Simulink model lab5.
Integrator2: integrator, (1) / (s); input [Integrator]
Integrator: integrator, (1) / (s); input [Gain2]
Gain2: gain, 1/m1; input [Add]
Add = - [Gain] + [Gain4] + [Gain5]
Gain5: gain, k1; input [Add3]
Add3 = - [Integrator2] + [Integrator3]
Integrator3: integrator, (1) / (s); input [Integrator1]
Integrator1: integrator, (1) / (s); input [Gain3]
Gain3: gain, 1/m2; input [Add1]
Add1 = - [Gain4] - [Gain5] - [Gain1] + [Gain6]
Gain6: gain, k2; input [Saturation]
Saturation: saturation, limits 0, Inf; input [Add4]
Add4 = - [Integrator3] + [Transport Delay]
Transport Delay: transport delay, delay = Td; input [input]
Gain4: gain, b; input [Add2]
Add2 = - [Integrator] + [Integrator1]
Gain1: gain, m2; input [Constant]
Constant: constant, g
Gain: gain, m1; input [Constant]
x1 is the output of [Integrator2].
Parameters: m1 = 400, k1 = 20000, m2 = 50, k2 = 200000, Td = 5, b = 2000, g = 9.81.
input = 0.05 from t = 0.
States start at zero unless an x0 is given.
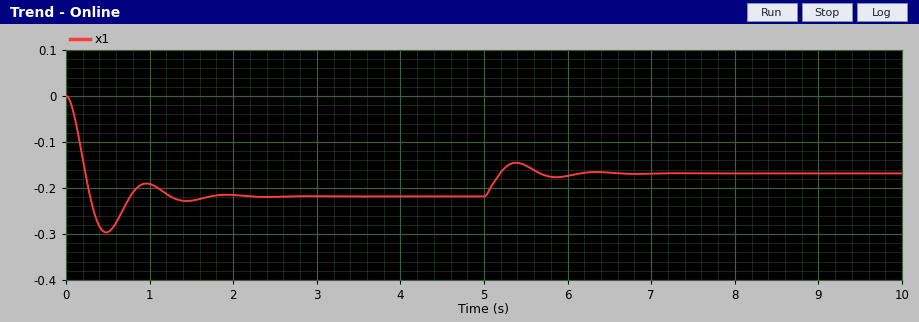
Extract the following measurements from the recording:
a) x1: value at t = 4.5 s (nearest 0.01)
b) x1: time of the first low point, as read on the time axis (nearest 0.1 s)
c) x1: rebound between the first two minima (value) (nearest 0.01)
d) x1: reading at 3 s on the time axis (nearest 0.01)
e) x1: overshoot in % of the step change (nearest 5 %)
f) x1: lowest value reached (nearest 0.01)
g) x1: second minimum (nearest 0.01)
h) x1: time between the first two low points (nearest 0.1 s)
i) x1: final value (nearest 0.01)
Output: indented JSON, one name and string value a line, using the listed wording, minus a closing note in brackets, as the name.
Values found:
{
  "x1: value at t = 4.5 s": "-0.22",
  "x1: time of the first low point, as read on the time axis": "0.5 s",
  "x1: rebound between the first two minima (value)": "-0.19",
  "x1: reading at 3 s on the time axis": "-0.22",
  "x1: overshoot in % of the step change": "75 %",
  "x1: lowest value reached": "-0.30",
  "x1: second minimum": "-0.23",
  "x1: time between the first two low points": "1.0 s",
  "x1: final value": "-0.17"
}
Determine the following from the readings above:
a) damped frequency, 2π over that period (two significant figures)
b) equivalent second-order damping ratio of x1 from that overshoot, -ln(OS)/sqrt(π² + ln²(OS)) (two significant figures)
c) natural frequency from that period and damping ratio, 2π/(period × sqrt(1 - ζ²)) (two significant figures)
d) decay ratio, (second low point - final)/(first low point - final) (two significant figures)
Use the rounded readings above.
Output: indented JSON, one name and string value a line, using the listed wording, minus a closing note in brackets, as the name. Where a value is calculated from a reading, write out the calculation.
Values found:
{
  "damped frequency, 2π over that period": "2π / 1 = 6.3 rad/s",
  "equivalent second-order damping ratio of x1 from that overshoot, -ln(OS)/sqrt(π² + ln²(OS))": "ln(0.75) = -0.288; 0.288 / sqrt(9.870 + 0.083) = 0.091",
  "natural frequency from that period and damping ratio, 2π/(period × sqrt(1 - ζ²))": "2π / (1 × sqrt(1 - 0.091²)) = 6.3 rad/s",
  "decay ratio, (second low point - final)/(first low point - final)": "(-0.23 - (-0.17)) / (-0.3 - (-0.17)) = 0.46"
}
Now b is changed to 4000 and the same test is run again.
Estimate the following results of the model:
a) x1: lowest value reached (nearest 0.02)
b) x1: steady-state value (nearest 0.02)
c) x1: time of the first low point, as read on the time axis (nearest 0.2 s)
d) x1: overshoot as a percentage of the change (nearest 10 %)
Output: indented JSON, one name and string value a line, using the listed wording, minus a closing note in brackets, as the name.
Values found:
{
  "x1: lowest value reached": "-0.24",
  "x1: steady-state value": "-0.16",
  "x1: time of the first low point, as read on the time axis": "0.6 s",
  "x1: overshoot as a percentage of the change": "40 %"
}
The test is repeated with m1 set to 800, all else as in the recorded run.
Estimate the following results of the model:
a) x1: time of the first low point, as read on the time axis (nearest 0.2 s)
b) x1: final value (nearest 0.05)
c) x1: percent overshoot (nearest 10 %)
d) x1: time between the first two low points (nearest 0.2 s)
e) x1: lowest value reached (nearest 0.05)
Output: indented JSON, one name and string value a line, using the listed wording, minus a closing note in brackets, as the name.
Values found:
{
  "x1: time of the first low point, as read on the time axis": "0.6 s",
  "x1: final value": "-0.40",
  "x1: percent overshoot": "70 %",
  "x1: time between the first two low points": "1.4 s",
  "x1: lowest value reached": "-0.65"
}
